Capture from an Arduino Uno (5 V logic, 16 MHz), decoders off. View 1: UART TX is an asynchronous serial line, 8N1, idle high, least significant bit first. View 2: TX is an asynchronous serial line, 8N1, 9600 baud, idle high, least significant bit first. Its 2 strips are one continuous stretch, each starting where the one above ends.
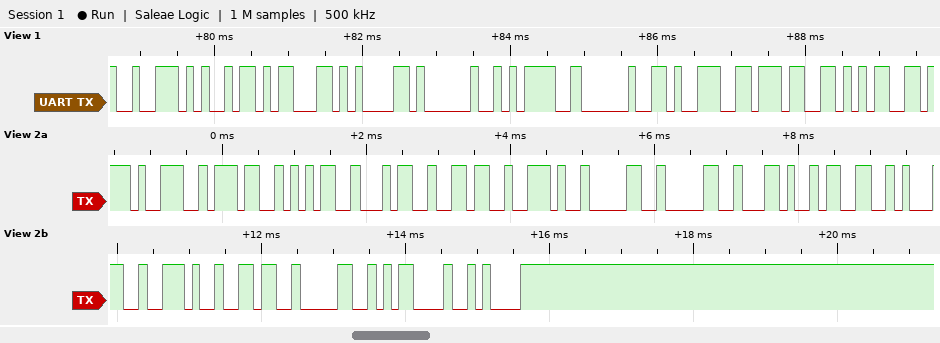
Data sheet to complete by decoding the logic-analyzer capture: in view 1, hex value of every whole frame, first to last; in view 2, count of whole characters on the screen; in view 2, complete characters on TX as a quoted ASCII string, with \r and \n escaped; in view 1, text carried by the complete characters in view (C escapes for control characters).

0x72 0x69 0x63 0x61 0x20 0x3D 0x20 0x39 0x37 0x35
16
"97546.00,31.60\r\n"
"rica = 975"
